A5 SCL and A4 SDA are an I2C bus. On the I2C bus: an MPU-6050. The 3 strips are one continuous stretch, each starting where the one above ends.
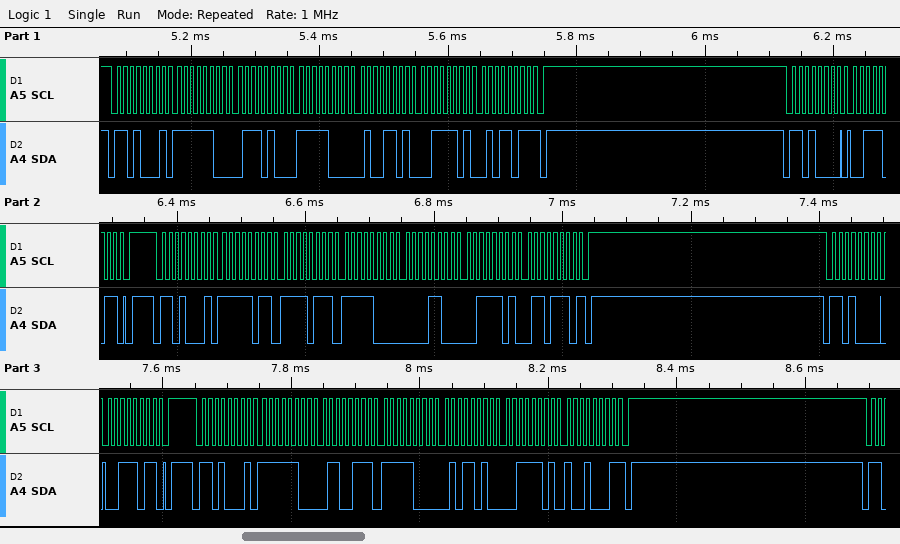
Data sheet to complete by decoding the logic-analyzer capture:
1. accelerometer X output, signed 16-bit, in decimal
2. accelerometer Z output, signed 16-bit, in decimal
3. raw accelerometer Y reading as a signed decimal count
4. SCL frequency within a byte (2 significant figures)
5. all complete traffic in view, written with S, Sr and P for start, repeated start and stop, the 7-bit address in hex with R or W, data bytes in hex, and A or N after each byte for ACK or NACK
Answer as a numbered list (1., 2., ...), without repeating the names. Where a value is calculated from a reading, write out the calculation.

1. 0xFBF7 = -1033
2. 0x3D6E = 15726
3. 0xF80C = -2036
4. 100 kHz
5. S 68R A FC A 74 A F8 A 4D A 3D A 5B N P S 68W A 3B A P S 68R A FB A F7 A F8 A 0C A 3D A 6E N P S 68W A 3B A P S 68R A FC A 67 A F8 A 5A A 3D A 91 N P
